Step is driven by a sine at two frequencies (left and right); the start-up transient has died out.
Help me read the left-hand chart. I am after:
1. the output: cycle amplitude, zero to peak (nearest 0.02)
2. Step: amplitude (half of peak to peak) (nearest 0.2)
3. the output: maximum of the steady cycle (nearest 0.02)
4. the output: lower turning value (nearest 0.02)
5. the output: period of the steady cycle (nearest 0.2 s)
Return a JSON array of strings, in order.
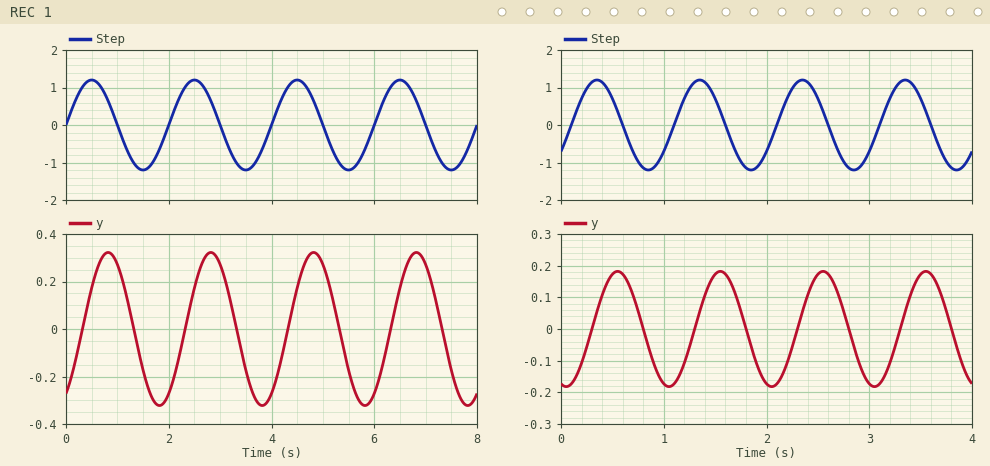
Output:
["0.32", "1.2", "0.32", "-0.32", "2.0 s"]
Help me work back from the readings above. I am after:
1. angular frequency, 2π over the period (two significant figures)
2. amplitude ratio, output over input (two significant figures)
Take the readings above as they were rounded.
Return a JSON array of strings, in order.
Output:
["3.1 rad/s", "0.27"]
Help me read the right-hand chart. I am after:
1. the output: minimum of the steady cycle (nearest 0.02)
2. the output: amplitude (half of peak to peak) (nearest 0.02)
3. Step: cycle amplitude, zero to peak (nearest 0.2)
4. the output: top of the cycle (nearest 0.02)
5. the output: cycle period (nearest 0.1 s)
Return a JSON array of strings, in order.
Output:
["-0.18", "0.18", "1.2", "0.18", "1.0 s"]
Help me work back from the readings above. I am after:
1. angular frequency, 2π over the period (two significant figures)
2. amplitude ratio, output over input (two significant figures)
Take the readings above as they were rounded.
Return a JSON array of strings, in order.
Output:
["6.3 rad/s", "0.15"]
